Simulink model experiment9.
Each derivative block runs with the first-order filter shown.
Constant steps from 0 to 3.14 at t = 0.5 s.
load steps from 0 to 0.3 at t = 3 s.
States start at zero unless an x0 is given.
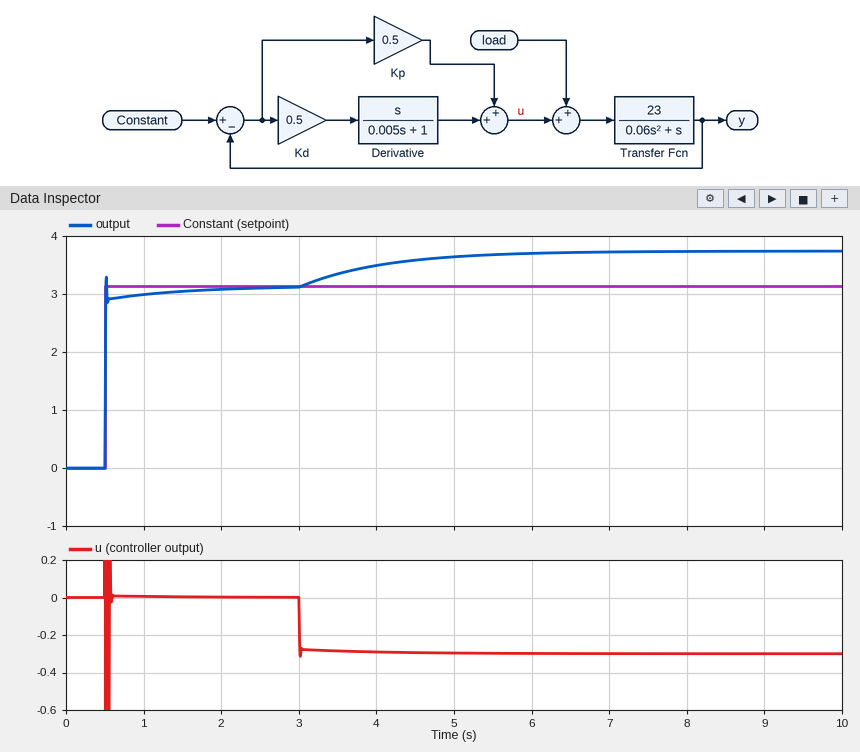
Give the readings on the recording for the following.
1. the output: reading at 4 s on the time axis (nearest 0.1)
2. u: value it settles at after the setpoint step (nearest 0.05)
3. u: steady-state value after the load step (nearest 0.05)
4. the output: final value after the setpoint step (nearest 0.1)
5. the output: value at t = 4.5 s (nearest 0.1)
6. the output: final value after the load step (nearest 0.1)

3.5
0.00
-0.30
3.1
3.6
3.7
